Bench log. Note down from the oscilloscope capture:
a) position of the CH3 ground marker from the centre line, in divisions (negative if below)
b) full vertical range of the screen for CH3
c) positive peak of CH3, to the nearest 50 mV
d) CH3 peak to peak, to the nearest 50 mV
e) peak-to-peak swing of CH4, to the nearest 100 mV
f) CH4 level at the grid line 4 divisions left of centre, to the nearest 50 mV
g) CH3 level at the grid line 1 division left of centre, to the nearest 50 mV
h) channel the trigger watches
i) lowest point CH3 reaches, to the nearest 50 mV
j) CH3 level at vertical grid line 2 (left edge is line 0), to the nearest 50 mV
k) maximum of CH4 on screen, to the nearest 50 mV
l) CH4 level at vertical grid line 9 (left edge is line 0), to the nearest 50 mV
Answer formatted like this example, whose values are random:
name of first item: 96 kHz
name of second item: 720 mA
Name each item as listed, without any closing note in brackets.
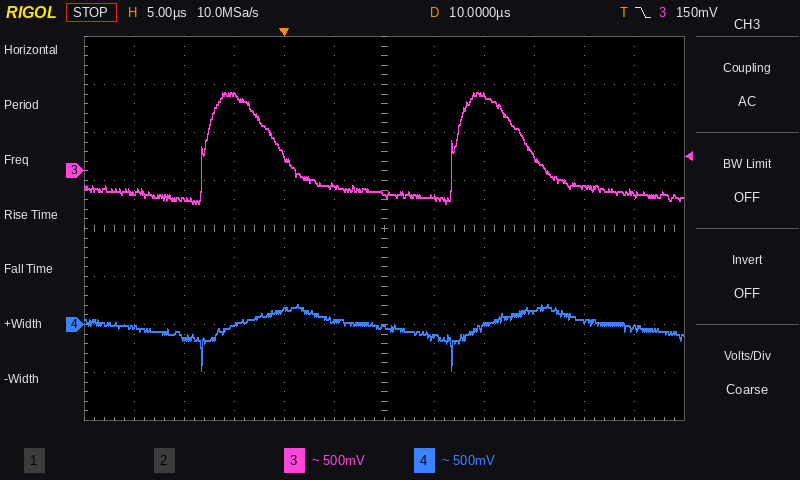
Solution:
position of the CH3 ground marker from the centre line, in divisions: +1.2 div
full vertical range of the screen for CH3: 4 V
positive peak of CH3, to the nearest 50 mV: 800 mV
CH3 peak to peak, to the nearest 50 mV: 1.15 V
peak-to-peak swing of CH4, to the nearest 100 mV: 700 mV
CH4 level at the grid line 4 divisions left of centre, to the nearest 50 mV: -150 mV
CH3 level at the grid line 1 division left of centre, to the nearest 50 mV: -150 mV
channel the trigger watches: CH3
lowest point CH3 reaches, to the nearest 50 mV: -350 mV
CH3 level at vertical grid line 2 (left edge is line 0), to the nearest 50 mV: -300 mV
maximum of CH4 on screen, to the nearest 50 mV: 200 mV
CH4 level at vertical grid line 9 (left edge is line 0), to the nearest 50 mV: 150 mV
